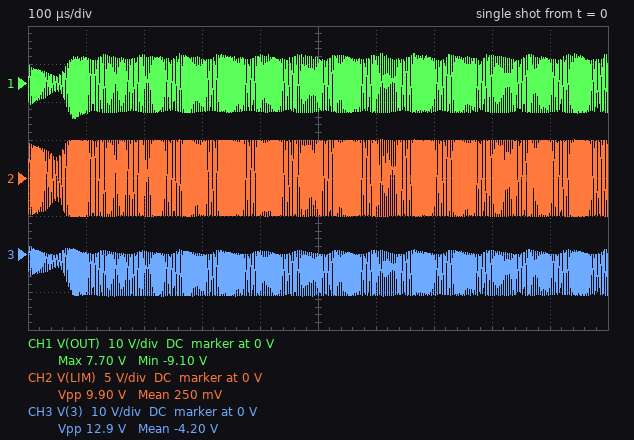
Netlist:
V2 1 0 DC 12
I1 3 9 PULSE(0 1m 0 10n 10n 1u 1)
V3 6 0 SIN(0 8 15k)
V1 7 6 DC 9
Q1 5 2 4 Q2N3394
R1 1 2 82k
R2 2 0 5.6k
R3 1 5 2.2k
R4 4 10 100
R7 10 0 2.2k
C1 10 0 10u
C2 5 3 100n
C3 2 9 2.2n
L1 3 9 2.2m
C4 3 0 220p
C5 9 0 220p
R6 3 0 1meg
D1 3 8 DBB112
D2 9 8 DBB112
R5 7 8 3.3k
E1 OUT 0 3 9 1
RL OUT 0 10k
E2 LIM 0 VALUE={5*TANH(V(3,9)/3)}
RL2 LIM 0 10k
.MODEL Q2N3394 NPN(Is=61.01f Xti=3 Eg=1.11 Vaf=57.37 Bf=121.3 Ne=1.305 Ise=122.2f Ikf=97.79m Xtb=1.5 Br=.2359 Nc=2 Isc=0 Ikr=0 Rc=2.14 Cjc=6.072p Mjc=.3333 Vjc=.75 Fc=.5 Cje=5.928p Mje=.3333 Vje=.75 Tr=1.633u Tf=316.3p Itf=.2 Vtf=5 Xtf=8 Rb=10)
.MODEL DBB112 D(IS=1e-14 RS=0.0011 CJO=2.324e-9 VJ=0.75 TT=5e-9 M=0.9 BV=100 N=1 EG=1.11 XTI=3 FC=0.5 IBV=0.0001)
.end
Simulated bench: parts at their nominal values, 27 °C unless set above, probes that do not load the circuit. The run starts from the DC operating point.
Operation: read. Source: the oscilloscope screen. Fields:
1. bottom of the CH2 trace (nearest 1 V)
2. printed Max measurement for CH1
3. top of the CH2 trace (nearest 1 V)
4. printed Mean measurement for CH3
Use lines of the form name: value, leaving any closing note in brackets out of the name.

bottom of the CH2 trace: -5 V
printed Max measurement for CH1: 7.70 V
top of the CH2 trace: 5 V
printed Mean measurement for CH3: -4.20 V
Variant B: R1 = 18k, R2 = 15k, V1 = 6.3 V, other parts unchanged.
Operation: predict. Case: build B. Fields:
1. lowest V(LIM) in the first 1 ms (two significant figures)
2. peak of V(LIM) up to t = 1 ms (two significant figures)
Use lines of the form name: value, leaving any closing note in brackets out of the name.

lowest V(LIM) in the first 1 ms: -4.5 V
peak of V(LIM) up to t = 1 ms: 4.8 V
